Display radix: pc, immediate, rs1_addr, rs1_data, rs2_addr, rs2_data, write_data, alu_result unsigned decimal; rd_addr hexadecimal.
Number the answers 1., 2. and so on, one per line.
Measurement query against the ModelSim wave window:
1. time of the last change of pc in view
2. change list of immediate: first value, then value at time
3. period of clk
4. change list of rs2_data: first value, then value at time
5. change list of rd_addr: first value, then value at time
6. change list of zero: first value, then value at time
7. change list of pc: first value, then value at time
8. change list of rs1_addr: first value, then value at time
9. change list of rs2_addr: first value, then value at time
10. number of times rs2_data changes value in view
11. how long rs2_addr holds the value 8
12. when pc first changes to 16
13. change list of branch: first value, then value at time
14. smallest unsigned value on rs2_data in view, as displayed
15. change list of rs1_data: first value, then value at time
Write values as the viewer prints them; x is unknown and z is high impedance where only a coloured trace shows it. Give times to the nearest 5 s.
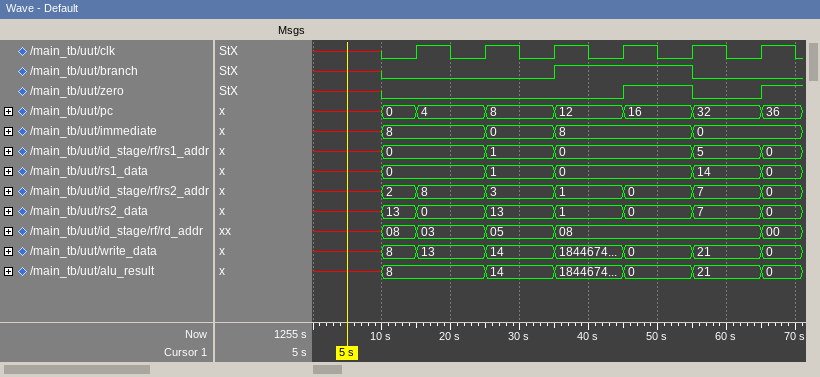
1. 65 s
2. x, 8 at 10 s, 0 at 25 s, 8 at 35 s, 0 at 55 s
3. 10 s
4. x, 13 at 10 s, 0 at 15 s, 13 at 25 s, 1 at 35 s, 0 at 45 s, 7 at 55 s, 0 at 65 s
5. x, 08 at 10 s, 03 at 15 s, 05 at 25 s, 08 at 35 s, 00 at 65 s
6. x, 0 at 10 s, 1 at 45 s, 0 at 55 s, 1 at 65 s
7. x, 0 at 10 s, 4 at 15 s, 8 at 25 s, 12 at 35 s, 16 at 45 s, 32 at 55 s, 36 at 65 s
8. x, 0 at 10 s, 1 at 25 s, 0 at 35 s, 5 at 55 s, 0 at 65 s
9. x, 2 at 10 s, 8 at 15 s, 3 at 25 s, 1 at 35 s, 0 at 45 s, 7 at 55 s, 0 at 65 s
10. 7
11. 10 s
12. 45 s
13. x, 0 at 10 s, 1 at 35 s, 0 at 55 s
14. 0
15. x, 0 at 10 s, 1 at 25 s, 0 at 35 s, 14 at 55 s, 0 at 65 s
